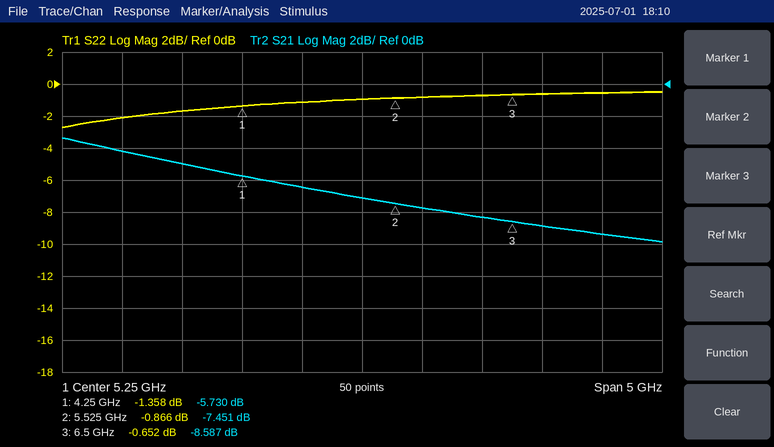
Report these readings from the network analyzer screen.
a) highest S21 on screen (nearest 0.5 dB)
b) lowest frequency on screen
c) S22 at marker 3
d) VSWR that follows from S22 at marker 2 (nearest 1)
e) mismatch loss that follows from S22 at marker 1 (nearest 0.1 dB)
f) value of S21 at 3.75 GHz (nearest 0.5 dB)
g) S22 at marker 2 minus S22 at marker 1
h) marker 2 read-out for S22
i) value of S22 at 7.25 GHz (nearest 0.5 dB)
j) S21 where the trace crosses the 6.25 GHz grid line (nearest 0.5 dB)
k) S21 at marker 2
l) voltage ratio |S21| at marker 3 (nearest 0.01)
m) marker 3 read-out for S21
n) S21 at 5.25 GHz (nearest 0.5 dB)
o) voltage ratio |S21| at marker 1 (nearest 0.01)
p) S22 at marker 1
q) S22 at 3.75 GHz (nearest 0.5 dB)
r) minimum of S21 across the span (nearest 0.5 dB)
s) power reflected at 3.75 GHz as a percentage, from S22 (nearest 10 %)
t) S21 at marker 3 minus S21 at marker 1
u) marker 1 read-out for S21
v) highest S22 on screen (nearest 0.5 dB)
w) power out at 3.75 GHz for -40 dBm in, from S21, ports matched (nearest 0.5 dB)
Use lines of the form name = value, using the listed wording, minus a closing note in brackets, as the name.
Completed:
highest S21 on screen = -3.5 dB
lowest frequency on screen = 2.75 GHz
S22 at marker 3 = -0.652 dB
VSWR that follows from S22 at marker 2 = 20
mismatch loss that follows from S22 at marker 1 = 5.7 dB
value of S21 at 3.75 GHz = -5.0 dB
S22 at marker 2 minus S22 at marker 1 = 0.492 dB
marker 2 read-out for S22 = -0.866 dB
value of S22 at 7.25 GHz = -0.5 dB
S21 where the trace crosses the 6.25 GHz grid line = -8.5 dB
S21 at marker 2 = -7.451 dB
voltage ratio |S21| at marker 3 = 0.37
marker 3 read-out for S21 = -8.587 dB
S21 at 5.25 GHz = -7.0 dB
voltage ratio |S21| at marker 1 = 0.52
S22 at marker 1 = -1.358 dB
S22 at 3.75 GHz = -1.5 dB
minimum of S21 across the span = -10.0 dB
power reflected at 3.75 GHz as a percentage, from S22 = 70 %
S21 at marker 3 minus S21 at marker 1 = -2.857 dB
marker 1 read-out for S21 = -5.730 dB
highest S22 on screen = -0.5 dB
power out at 3.75 GHz for -40 dBm in, from S21, ports matched = -45.0 dBm
